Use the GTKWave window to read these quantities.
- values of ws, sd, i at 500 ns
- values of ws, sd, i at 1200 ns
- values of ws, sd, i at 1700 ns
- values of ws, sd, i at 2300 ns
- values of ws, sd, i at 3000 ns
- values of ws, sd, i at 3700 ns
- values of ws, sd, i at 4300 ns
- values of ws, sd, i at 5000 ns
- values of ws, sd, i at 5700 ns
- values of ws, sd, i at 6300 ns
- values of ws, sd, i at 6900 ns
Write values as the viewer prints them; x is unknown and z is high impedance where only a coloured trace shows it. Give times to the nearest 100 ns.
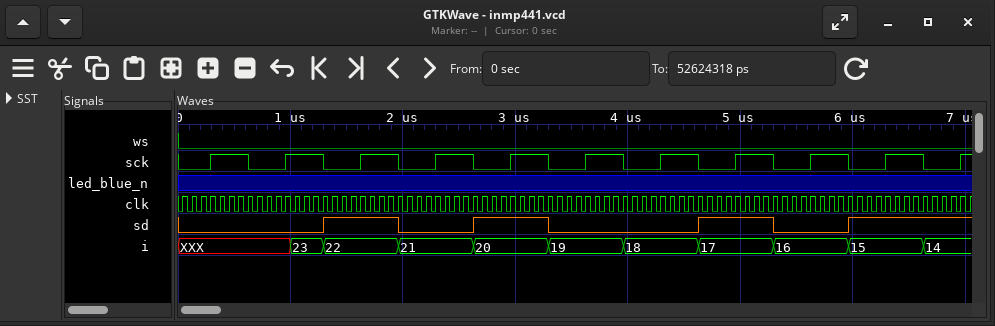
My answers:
ws=0, sd=0, i=XXX
ws=0, sd=0, i=23
ws=0, sd=1, i=22
ws=0, sd=0, i=21
ws=0, sd=1, i=20
ws=0, sd=0, i=19
ws=0, sd=0, i=18
ws=0, sd=1, i=17
ws=0, sd=0, i=16
ws=0, sd=1, i=15
ws=0, sd=1, i=14
